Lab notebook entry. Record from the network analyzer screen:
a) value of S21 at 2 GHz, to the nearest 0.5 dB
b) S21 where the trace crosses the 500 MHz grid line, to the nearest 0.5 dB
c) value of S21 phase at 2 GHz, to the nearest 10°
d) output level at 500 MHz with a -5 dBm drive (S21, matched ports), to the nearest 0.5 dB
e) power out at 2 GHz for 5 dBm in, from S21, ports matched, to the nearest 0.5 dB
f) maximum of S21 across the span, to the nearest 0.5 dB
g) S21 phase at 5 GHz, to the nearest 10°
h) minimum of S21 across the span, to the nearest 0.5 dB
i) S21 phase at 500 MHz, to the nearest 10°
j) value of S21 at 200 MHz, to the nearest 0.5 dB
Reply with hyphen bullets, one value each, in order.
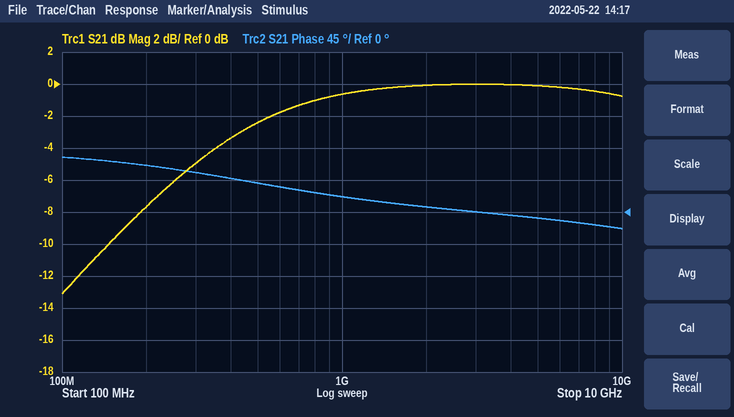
- 0.0 dB
- -2.5 dB
- 10°
- -7.5 dBm
- 5.0 dBm
- 0.0 dB
- -10°
- -13.0 dB
- 40°
- -7.5 dB
